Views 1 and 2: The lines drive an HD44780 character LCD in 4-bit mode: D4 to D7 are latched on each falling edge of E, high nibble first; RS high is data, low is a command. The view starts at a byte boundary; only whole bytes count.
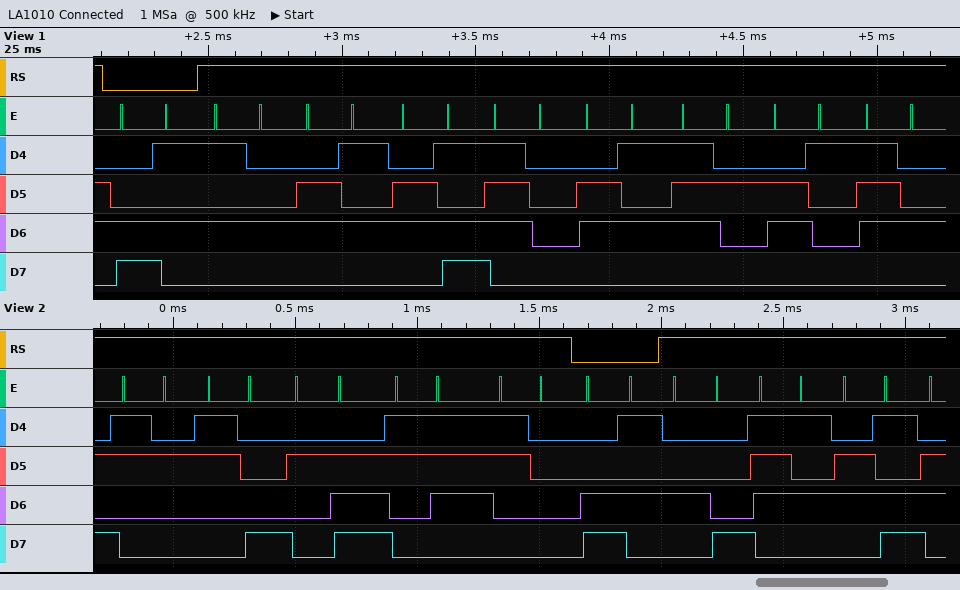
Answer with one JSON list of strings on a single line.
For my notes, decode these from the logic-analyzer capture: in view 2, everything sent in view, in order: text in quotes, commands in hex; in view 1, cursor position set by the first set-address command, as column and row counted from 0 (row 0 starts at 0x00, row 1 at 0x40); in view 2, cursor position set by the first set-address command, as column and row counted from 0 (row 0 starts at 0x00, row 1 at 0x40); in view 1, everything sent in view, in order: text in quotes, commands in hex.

["\"28.70\" 0xC5 \"Hum\"", "column 5, row 1", "column 5, row 1", "0xC5 \"Temperat\""]
